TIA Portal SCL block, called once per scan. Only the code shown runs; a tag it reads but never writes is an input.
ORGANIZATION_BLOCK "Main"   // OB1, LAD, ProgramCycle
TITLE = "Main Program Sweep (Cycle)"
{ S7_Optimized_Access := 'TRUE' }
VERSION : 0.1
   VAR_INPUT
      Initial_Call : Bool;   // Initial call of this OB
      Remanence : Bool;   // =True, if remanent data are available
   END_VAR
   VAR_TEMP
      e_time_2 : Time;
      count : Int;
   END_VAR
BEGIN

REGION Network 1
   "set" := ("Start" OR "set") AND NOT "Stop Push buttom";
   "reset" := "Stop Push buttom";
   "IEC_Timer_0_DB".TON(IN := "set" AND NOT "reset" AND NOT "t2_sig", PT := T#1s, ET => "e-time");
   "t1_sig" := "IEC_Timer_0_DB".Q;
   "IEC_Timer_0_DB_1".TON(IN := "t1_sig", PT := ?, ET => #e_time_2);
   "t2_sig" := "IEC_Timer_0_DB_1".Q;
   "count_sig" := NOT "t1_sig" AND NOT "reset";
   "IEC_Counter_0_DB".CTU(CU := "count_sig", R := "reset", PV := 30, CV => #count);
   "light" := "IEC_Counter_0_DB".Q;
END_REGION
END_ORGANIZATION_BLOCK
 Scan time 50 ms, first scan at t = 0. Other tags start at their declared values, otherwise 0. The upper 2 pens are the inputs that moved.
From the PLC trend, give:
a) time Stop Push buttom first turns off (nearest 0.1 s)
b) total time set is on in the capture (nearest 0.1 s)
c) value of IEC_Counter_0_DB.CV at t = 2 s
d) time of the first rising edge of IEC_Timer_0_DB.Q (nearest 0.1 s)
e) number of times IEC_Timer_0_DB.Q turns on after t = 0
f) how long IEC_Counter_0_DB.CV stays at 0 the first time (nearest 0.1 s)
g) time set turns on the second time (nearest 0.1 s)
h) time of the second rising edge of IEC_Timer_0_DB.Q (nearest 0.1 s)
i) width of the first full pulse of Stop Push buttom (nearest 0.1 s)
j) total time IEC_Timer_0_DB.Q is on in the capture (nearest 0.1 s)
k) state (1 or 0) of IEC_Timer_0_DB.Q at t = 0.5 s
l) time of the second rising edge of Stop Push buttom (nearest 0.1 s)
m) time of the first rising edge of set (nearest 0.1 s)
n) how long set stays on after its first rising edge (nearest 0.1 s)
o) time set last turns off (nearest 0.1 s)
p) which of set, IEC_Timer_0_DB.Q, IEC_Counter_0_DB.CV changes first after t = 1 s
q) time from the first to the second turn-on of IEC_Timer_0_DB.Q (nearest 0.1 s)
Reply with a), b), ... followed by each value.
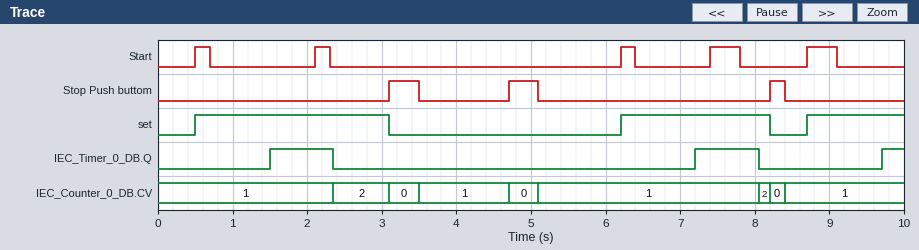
a) 3.5 s
b) 5.9 s
c) 1
d) 1.5 s
e) 3
f) 0.4 s
g) 6.2 s
h) 7.2 s
i) 0.4 s
j) 2.0 s
k) 0
l) 4.7 s
m) 0.5 s
n) 2.6 s
o) 8.2 s
p) IEC_Timer_0_DB.Q
q) 5.7 s
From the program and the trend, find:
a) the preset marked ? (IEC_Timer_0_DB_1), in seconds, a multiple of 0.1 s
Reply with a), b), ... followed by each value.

a) 0.8 s
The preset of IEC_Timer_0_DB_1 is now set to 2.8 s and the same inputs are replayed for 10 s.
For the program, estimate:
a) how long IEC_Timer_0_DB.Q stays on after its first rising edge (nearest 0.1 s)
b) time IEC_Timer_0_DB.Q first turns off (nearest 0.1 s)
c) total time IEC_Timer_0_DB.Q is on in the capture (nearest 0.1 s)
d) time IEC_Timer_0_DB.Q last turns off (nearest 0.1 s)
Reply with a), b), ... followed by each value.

a) 1.6 s
b) 3.1 s
c) 2.9 s
d) 8.2 s
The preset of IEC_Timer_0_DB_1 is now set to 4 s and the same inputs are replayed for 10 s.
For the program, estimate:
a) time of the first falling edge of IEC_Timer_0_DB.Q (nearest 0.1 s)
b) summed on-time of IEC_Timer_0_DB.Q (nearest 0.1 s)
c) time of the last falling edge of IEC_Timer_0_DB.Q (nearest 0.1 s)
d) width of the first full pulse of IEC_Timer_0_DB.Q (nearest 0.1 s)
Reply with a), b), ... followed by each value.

a) 3.1 s
b) 2.9 s
c) 8.2 s
d) 1.6 s
